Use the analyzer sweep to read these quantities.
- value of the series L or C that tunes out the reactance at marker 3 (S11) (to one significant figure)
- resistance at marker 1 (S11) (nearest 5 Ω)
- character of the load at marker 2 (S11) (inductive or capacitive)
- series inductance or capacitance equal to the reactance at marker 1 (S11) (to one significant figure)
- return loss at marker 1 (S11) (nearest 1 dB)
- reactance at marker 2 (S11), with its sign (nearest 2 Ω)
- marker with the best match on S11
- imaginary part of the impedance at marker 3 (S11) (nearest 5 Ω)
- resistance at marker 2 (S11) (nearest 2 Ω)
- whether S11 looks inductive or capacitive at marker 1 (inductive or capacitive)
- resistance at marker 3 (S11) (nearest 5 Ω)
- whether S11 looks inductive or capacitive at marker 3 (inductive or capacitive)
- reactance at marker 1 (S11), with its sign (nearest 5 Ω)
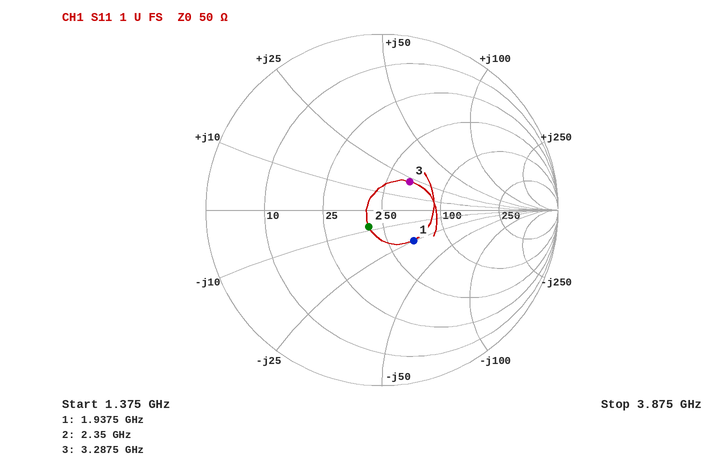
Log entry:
2 pF
65 Ω
capacitive
3 pF
12 dB
-8 Ω
marker 2
+20 Ω
42 Ω
capacitive
65 Ω
inductive
-25 Ω
